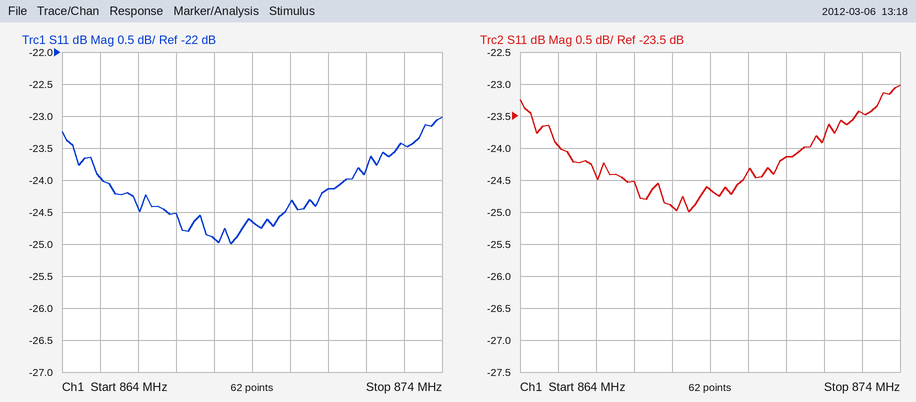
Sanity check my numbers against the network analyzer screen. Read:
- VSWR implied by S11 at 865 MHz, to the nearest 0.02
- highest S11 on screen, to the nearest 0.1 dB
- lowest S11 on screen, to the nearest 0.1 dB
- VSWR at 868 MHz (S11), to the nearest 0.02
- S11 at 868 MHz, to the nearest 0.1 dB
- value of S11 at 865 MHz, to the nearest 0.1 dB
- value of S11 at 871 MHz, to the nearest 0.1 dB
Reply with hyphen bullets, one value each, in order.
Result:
- 1.14
- -23.0 dB
- -25.0 dB
- 1.12
- -24.9 dB
- -24.0 dB
- -24.1 dB
